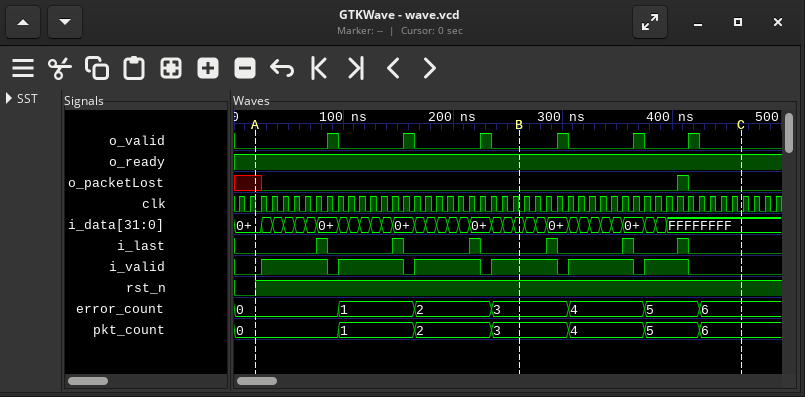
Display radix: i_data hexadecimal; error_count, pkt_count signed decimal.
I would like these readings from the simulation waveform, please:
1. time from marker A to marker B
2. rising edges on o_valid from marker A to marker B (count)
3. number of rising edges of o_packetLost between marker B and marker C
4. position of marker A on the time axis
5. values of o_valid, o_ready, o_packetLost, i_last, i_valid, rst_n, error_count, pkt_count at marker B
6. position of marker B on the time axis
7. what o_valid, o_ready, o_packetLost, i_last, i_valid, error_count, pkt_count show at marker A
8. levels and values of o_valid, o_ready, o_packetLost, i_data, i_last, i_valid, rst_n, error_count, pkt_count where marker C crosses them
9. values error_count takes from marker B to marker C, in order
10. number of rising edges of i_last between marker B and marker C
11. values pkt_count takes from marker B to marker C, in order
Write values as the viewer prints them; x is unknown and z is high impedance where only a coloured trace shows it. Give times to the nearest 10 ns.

240 ns
3
1
20 ns
o_valid=0, o_ready=1, o_packetLost=0, i_last=0, i_valid=1, rst_n=1, error_count=3, pkt_count=3
260 ns
o_valid=0, o_ready=1, o_packetLost=x, i_last=0, i_valid=0, error_count=0, pkt_count=0
o_valid=0, o_ready=1, o_packetLost=0, i_data=FFFFFFFF, i_last=0, i_valid=0, rst_n=1, error_count=6, pkt_count=6
3, 4, 5, 6
3
3, 4, 5, 6
